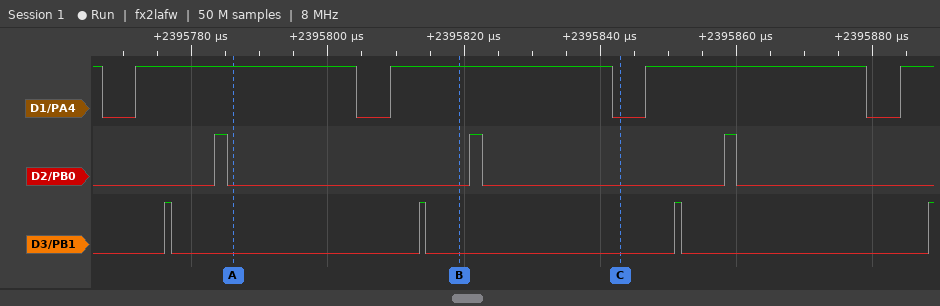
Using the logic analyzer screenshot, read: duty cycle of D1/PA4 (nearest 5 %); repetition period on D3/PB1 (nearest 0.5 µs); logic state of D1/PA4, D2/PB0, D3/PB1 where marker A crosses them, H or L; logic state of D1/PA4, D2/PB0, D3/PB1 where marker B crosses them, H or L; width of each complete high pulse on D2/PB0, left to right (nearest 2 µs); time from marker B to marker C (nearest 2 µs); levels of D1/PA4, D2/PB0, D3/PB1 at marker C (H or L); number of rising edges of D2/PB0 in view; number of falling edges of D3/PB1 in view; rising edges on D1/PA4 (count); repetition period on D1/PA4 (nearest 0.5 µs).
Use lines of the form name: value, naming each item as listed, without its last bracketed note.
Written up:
duty cycle of D1/PA4: 85 %
repetition period on D3/PB1: 37.5 µs
logic state of D1/PA4, D2/PB0, D3/PB1 where marker A crosses them, H or L: D1/PA4=H, D2/PB0=L, D3/PB1=L
logic state of D1/PA4, D2/PB0, D3/PB1 where marker B crosses them, H or L: D1/PA4=H, D2/PB0=L, D3/PB1=L
width of each complete high pulse on D2/PB0, left to right: 2 µs, 2 µs, 2 µs
time from marker B to marker C: 24 µs
levels of D1/PA4, D2/PB0, D3/PB1 at marker C: D1/PA4=L, D2/PB0=L, D3/PB1=L
number of rising edges of D2/PB0 in view: 3
number of falling edges of D3/PB1 in view: 3
rising edges on D1/PA4: 4
repetition period on D1/PA4: 37.5 µs
